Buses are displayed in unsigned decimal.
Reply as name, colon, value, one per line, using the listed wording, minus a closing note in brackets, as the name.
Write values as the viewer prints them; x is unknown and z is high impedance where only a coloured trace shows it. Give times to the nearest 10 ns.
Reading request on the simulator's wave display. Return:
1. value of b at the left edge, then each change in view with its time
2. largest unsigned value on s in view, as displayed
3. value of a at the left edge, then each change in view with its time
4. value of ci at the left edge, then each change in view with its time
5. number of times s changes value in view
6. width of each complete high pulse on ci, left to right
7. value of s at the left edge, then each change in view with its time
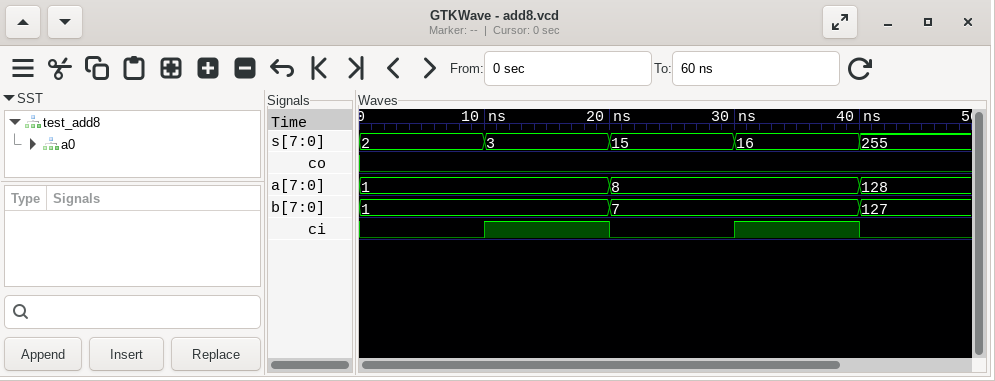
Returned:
value of b at the left edge, then each change in view with its time: 1, 7 at 20 ns, 127 at 40 ns
largest unsigned value on s in view, as displayed: 255
value of a at the left edge, then each change in view with its time: 1, 8 at 20 ns, 128 at 40 ns
value of ci at the left edge, then each change in view with its time: 0, 1 at 10 ns, 0 at 20 ns, 1 at 30 ns, 0 at 40 ns
number of times s changes value in view: 4
width of each complete high pulse on ci, left to right: 10 ns, 10 ns
value of s at the left edge, then each change in view with its time: 2, 3 at 10 ns, 15 at 20 ns, 16 at 30 ns, 255 at 40 ns
